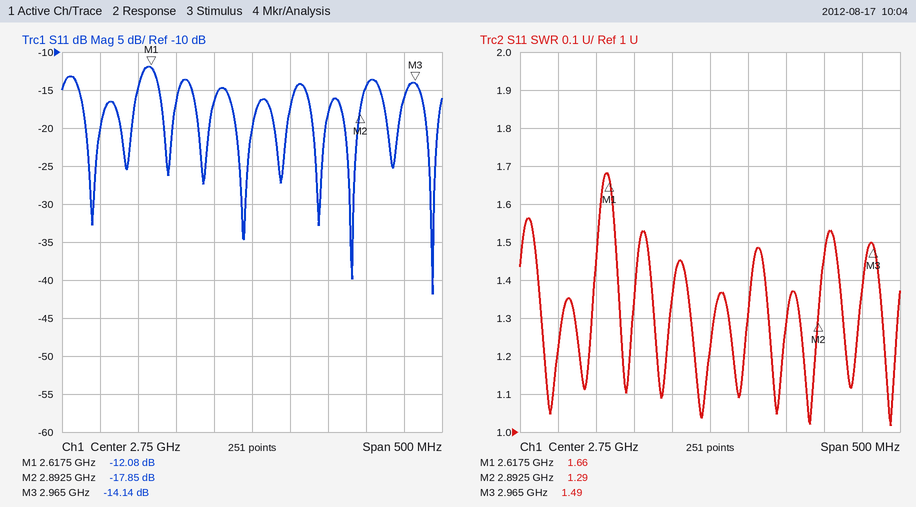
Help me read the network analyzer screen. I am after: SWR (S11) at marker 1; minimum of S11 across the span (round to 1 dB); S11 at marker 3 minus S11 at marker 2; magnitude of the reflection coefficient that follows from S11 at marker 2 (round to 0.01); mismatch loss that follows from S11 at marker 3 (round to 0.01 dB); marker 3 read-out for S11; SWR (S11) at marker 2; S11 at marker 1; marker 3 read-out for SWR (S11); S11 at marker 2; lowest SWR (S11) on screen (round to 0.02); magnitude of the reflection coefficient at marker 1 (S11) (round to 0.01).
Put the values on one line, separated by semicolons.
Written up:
1.66; -42 dB; 3.71 dB; 0.13; 0.17 dB; -14.14 dB; 1.29; -12.08 dB; 1.49; -17.85 dB; 1.02; 0.25
